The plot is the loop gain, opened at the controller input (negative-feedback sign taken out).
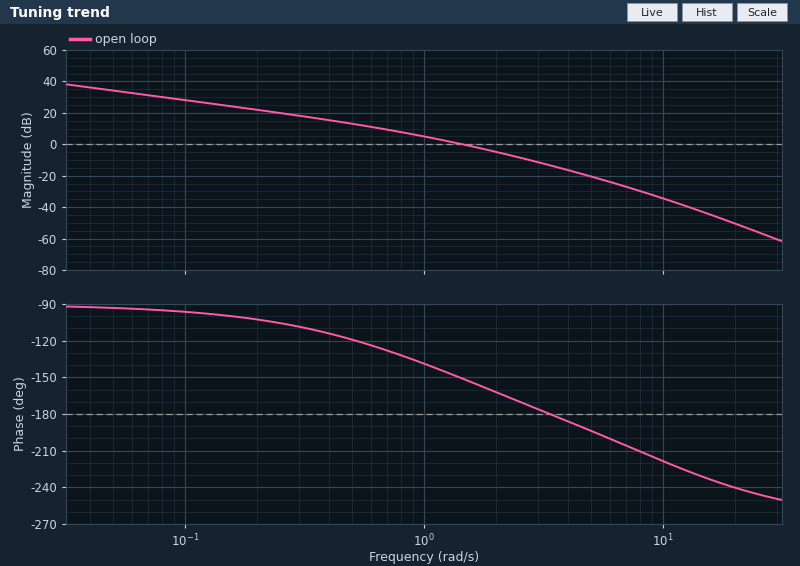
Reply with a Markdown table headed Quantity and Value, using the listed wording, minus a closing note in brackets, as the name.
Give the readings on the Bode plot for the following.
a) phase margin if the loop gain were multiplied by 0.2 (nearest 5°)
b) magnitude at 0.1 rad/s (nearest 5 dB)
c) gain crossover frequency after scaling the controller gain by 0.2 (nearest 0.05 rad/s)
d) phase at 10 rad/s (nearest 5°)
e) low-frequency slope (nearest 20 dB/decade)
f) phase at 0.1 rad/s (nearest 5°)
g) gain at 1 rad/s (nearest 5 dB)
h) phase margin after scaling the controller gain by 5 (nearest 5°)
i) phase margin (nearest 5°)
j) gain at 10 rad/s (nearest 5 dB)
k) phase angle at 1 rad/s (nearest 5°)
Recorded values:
| Quantity | Value |
|---|---|
| phase margin if the loop gain were multiplied by 0.2 | 65° |
| magnitude at 0.1 rad/s | 30 dB |
| gain crossover frequency after scaling the controller gain by 0.2 | 0.45 rad/s |
| phase at 10 rad/s | -220° |
| low-frequency slope | -20 dB/decade |
| phase at 0.1 rad/s | -95° |
| gain at 1 rad/s | 5 dB |
| phase margin after scaling the controller gain by 5 | 0° |
| phase margin | 30° |
| gain at 10 rad/s | -35 dB |
| phase angle at 1 rad/s | -140° |
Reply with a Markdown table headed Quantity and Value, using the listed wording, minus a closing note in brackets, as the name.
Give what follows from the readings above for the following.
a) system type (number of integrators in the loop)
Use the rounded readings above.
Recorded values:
| Quantity | Value |
|---|---|
| system type | 1 |
